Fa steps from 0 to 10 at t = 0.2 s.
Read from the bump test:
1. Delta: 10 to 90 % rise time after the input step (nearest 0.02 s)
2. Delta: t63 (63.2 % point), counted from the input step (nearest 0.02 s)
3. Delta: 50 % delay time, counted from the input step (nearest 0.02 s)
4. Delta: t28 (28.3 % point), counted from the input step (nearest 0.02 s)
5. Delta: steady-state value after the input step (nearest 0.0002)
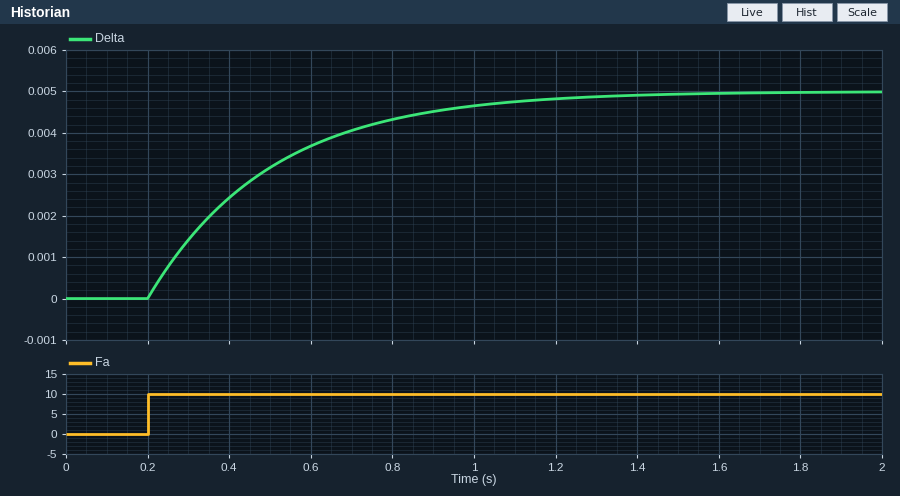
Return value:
0.66 s
0.30 s
0.20 s
0.10 s
0.0050
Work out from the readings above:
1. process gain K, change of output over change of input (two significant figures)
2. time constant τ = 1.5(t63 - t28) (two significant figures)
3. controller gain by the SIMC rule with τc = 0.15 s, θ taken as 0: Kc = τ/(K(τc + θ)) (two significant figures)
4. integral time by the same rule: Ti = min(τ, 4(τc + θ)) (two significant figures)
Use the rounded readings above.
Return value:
0.00050
0.30 s
4000
0.30 s
